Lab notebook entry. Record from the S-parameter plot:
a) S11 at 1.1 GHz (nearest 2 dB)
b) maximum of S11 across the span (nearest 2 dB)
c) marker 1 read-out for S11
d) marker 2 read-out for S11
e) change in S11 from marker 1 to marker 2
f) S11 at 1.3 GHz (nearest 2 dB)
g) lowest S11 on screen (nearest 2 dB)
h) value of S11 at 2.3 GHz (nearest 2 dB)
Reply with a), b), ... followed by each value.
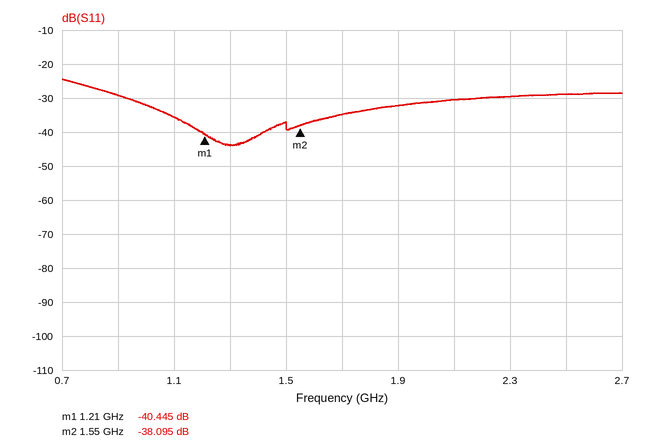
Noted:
a) -36 dB
b) -24 dB
c) -40.445 dB
d) -38.095 dB
e) 2.350 dB
f) -44 dB
g) -44 dB
h) -30 dB
